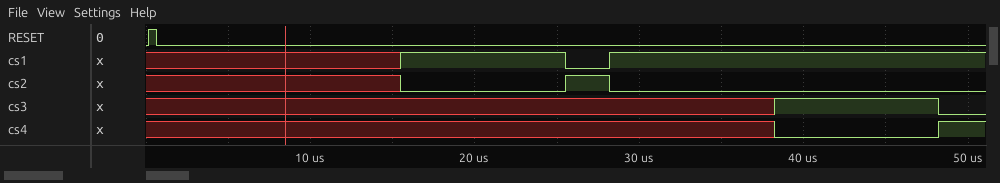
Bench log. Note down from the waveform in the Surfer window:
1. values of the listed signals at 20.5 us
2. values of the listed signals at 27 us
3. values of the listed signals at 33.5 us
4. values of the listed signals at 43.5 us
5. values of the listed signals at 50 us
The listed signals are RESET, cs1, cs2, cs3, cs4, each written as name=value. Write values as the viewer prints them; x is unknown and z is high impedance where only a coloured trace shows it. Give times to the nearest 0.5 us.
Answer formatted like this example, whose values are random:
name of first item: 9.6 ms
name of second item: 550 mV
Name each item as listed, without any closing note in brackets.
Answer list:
values of the listed signals at 20.5 us: RESET=0, cs1=1, cs2=0, cs3=x, cs4=x
values of the listed signals at 27 us: RESET=0, cs1=0, cs2=1, cs3=x, cs4=x
values of the listed signals at 33.5 us: RESET=0, cs1=1, cs2=0, cs3=x, cs4=x
values of the listed signals at 43.5 us: RESET=0, cs1=1, cs2=0, cs3=1, cs4=0
values of the listed signals at 50 us: RESET=0, cs1=1, cs2=0, cs3=0, cs4=1
